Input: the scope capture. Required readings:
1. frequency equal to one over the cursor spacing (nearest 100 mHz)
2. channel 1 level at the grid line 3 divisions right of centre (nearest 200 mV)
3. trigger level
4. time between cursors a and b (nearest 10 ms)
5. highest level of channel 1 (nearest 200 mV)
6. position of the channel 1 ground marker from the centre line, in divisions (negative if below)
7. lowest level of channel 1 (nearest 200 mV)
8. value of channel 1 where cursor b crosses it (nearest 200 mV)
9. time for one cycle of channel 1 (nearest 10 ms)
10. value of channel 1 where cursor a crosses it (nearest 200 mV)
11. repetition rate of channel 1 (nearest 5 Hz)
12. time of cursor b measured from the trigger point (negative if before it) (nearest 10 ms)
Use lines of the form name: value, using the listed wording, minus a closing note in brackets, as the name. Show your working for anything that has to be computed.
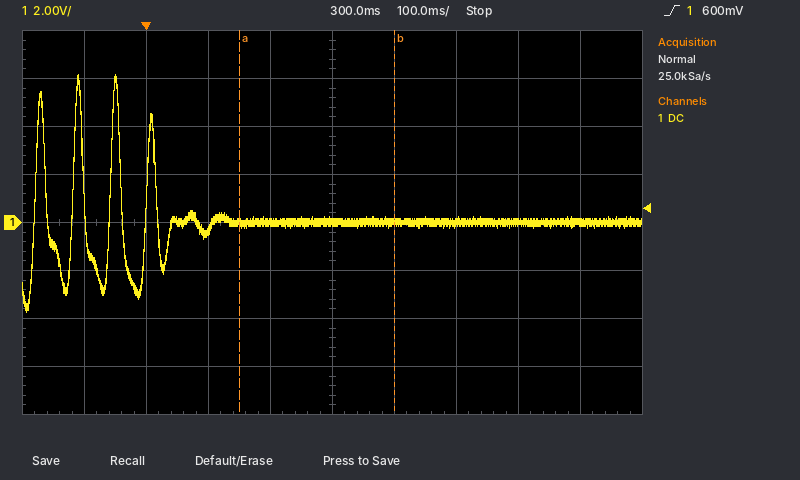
frequency equal to one over the cursor spacing: 1 / 250 ms ≈ 4.0 Hz
channel 1 level at the grid line 3 divisions right of centre: 0.0 V
trigger level: 600 mV
time between cursors a and b: 250 ms
highest level of channel 1: 6.2 V
position of the channel 1 ground marker from the centre line, in divisions: 0.0 div
lowest level of channel 1: -3.8 V
value of channel 1 where cursor b crosses it: 0.0 V
time for one cycle of channel 1: 60 ms
value of channel 1 where cursor a crosses it: 0.0 V
repetition rate of channel 1: 1 / 60 ms ≈ 16.7 Hz, so 15 Hz to the nearest 5 Hz
time of cursor b measured from the trigger point (negative if before it): +400 ms
